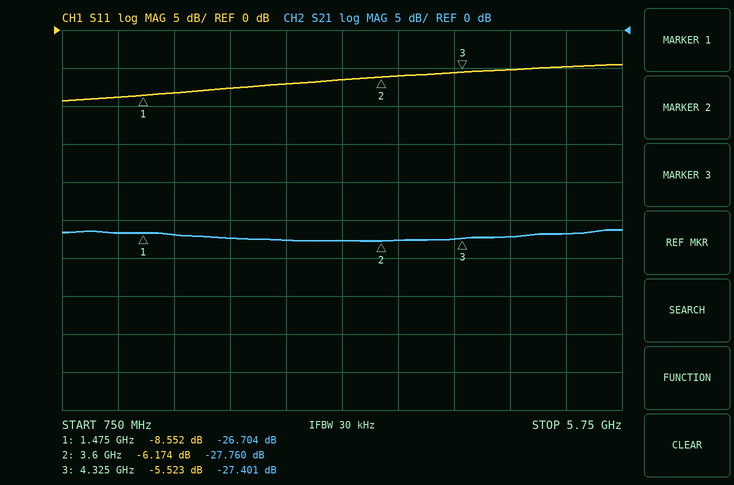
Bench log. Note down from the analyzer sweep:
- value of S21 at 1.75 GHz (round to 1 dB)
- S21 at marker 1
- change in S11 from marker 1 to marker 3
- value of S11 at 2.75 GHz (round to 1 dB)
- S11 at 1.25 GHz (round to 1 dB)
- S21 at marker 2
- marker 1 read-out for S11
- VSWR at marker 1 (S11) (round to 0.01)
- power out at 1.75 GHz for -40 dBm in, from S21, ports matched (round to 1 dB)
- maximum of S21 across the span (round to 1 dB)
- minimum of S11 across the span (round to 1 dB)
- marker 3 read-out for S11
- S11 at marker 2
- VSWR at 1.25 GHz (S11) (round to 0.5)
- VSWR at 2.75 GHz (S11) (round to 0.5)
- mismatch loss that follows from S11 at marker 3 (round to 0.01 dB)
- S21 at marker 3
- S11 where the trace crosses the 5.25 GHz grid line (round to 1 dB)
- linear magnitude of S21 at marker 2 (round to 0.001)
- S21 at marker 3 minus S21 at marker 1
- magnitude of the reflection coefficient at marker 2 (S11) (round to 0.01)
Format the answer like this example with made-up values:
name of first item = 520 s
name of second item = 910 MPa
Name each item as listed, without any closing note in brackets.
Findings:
value of S21 at 1.75 GHz = -27 dB
S21 at marker 1 = -26.704 dB
change in S11 from marker 1 to marker 3 = 3.029 dB
value of S11 at 2.75 GHz = -7 dB
S11 at 1.25 GHz = -9 dB
S21 at marker 2 = -27.760 dB
marker 1 read-out for S11 = -8.552 dB
VSWR at marker 1 (S11) = 2.19
power out at 1.75 GHz for -40 dBm in, from S21, ports matched = -67 dBm
maximum of S21 across the span = -26 dB
minimum of S11 across the span = -9 dB
marker 3 read-out for S11 = -5.523 dB
S11 at marker 2 = -6.174 dB
VSWR at 1.25 GHz (S11) = 2.0
VSWR at 2.75 GHz (S11) = 2.5
mismatch loss that follows from S11 at marker 3 = 1.43 dB
S21 at marker 3 = -27.401 dB
S11 where the trace crosses the 5.25 GHz grid line = -5 dB
linear magnitude of S21 at marker 2 = 0.041
S21 at marker 3 minus S21 at marker 1 = -0.697 dB
magnitude of the reflection coefficient at marker 2 (S11) = 0.49
